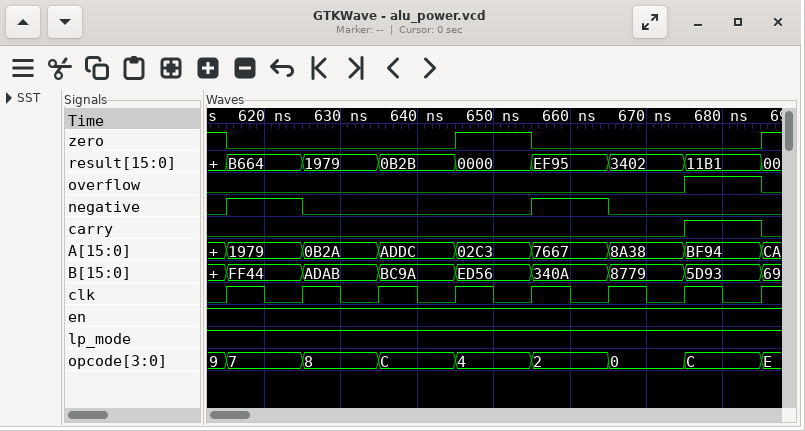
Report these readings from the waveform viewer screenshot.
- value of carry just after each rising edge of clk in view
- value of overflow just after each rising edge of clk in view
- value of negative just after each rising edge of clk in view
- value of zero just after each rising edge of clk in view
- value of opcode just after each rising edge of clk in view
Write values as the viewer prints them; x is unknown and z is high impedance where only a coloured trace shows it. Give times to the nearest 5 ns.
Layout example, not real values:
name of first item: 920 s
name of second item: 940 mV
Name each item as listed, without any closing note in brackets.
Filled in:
value of carry just after each rising edge of clk in view: 0 0 0 0 0 0 1 0
value of overflow just after each rising edge of clk in view: 0 0 0 0 0 0 1 0
value of negative just after each rising edge of clk in view: 1 0 0 0 1 0 0 0
value of zero just after each rising edge of clk in view: 0 0 0 1 0 0 0 1
value of opcode just after each rising edge of clk in view: 7, 8, C, 4, 2, 0, C, E
